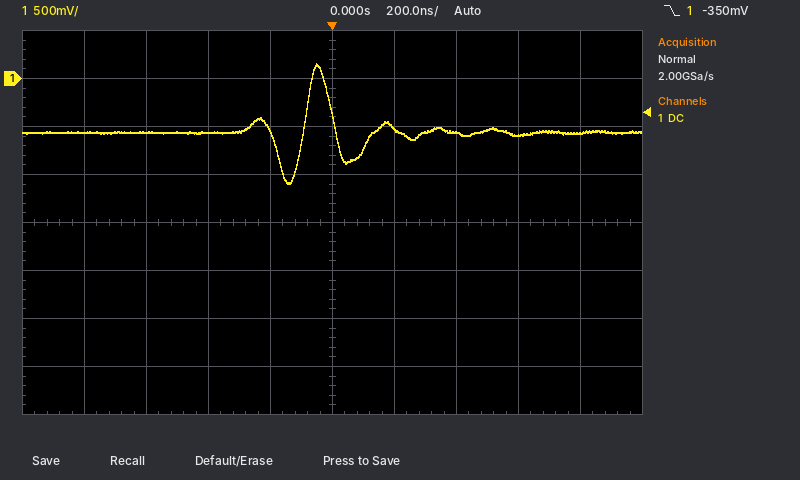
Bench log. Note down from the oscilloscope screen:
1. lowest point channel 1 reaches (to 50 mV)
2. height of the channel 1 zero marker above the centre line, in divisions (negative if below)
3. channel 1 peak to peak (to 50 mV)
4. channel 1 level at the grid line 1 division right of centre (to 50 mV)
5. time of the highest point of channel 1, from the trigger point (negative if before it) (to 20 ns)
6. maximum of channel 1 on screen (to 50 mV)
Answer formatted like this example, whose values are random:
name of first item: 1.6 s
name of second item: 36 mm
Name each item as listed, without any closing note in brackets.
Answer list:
lowest point channel 1 reaches: -1.10 V
height of the channel 1 zero marker above the centre line, in divisions: +3.0 div
channel 1 peak to peak: 1.25 V
channel 1 level at the grid line 1 division right of centre: -500 mV
time of the highest point of channel 1, from the trigger point (negative if before it): -40 ns
maximum of channel 1 on screen: 150 mV
